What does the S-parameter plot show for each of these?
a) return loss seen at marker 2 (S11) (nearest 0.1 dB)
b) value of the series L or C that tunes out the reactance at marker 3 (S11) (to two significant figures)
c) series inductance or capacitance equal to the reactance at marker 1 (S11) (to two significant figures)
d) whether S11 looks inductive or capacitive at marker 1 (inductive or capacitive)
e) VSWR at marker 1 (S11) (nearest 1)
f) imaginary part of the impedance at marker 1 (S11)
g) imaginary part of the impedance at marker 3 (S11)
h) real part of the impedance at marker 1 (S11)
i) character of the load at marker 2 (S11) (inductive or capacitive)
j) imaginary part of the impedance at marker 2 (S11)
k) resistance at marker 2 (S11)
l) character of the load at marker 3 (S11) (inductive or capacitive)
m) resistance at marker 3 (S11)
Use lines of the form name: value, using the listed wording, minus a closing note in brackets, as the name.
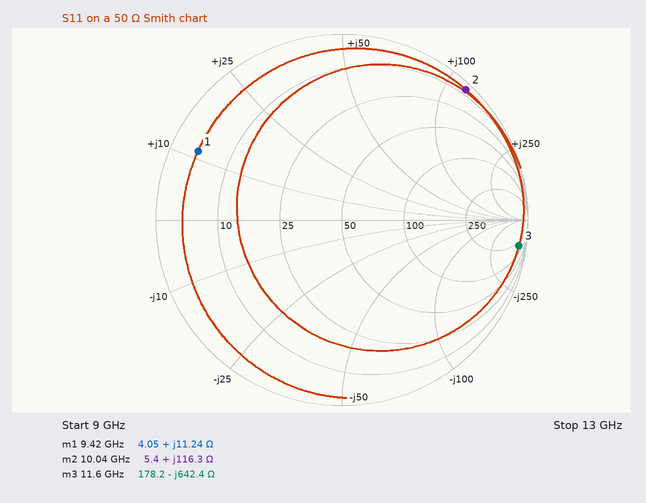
return loss seen at marker 2 (S11): 0.3 dB
value of the series L or C that tunes out the reactance at marker 3 (S11): 8.8 nH
series inductance or capacitance equal to the reactance at marker 1 (S11): 190 pH
whether S11 looks inductive or capacitive at marker 1: inductive
VSWR at marker 1 (S11): 13
imaginary part of the impedance at marker 1: +11.24 Ω
imaginary part of the impedance at marker 3: -642.4 Ω
real part of the impedance at marker 1: 4.05 Ω
character of the load at marker 2 (S11): inductive
imaginary part of the impedance at marker 2: +116.3 Ω
resistance at marker 2: 5.4 Ω
character of the load at marker 3 (S11): capacitive
resistance at marker 3: 178.2 Ω
